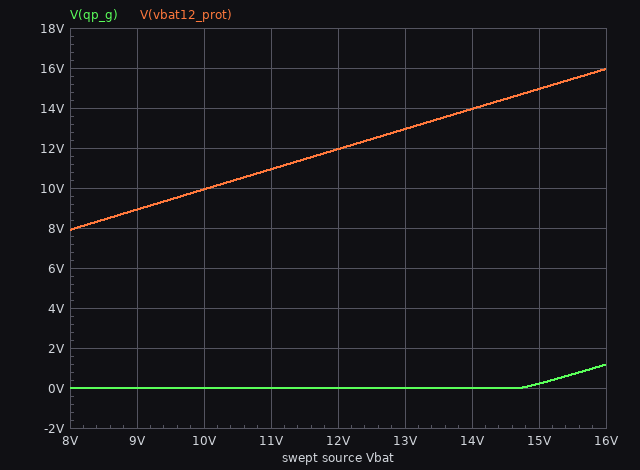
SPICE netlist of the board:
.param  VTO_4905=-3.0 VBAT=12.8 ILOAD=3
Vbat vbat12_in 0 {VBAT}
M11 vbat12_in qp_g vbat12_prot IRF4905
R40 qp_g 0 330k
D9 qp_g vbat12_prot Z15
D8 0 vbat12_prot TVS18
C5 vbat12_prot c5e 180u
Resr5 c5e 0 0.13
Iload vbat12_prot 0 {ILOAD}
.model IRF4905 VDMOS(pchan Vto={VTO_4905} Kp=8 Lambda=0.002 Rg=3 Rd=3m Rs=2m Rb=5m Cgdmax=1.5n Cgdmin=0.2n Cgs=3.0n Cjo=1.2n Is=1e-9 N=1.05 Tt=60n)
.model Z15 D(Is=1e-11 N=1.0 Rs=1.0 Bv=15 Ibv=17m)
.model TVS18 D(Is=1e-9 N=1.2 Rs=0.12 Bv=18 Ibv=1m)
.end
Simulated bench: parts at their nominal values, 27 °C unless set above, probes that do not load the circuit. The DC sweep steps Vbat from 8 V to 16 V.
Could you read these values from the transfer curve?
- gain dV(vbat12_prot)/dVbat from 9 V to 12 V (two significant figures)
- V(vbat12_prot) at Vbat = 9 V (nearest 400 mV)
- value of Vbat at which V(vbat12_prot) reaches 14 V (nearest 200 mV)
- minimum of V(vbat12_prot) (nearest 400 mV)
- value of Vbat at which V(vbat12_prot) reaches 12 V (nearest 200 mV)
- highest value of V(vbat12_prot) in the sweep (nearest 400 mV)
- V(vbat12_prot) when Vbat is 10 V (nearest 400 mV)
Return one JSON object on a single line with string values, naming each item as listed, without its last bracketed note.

{"gain dV(vbat12_prot)/dVbat from 9 V to 12 V": "1.0 V/V", "V(vbat12_prot) at Vbat = 9 V": "8.8 V", "value of Vbat at which V(vbat12_prot) reaches 14 V": "14.0 V", "minimum of V(vbat12_prot)": "8.0 V", "value of Vbat at which V(vbat12_prot) reaches 12 V": "12.0 V", "highest value of V(vbat12_prot) in the sweep": "16.0 V", "V(vbat12_prot) when Vbat is 10 V": "10.0 V"}
